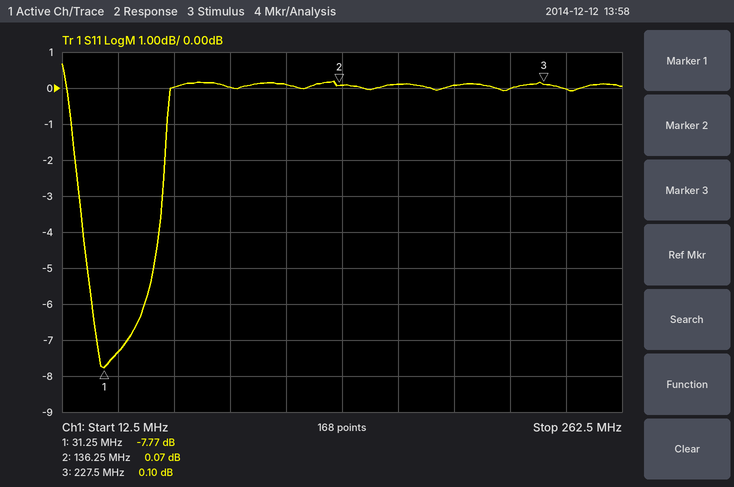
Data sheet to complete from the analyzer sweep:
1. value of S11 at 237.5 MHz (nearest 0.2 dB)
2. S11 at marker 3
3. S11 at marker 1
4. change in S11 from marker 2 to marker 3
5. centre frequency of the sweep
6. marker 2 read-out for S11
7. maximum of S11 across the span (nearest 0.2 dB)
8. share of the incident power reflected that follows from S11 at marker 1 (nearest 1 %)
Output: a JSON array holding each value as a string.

["0.0 dB", "0.10 dB", "-7.77 dB", "0.03 dB", "137.5 MHz", "0.07 dB", "0.6 dB", "17 %"]
